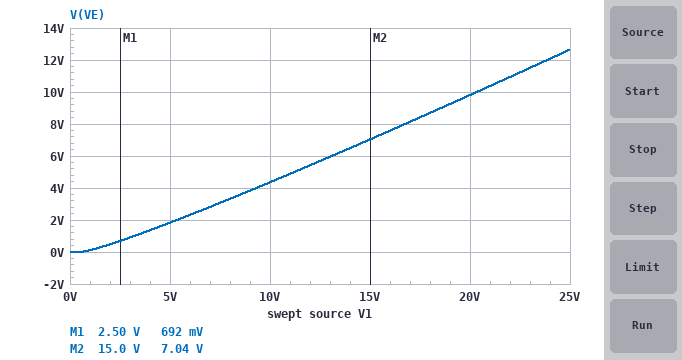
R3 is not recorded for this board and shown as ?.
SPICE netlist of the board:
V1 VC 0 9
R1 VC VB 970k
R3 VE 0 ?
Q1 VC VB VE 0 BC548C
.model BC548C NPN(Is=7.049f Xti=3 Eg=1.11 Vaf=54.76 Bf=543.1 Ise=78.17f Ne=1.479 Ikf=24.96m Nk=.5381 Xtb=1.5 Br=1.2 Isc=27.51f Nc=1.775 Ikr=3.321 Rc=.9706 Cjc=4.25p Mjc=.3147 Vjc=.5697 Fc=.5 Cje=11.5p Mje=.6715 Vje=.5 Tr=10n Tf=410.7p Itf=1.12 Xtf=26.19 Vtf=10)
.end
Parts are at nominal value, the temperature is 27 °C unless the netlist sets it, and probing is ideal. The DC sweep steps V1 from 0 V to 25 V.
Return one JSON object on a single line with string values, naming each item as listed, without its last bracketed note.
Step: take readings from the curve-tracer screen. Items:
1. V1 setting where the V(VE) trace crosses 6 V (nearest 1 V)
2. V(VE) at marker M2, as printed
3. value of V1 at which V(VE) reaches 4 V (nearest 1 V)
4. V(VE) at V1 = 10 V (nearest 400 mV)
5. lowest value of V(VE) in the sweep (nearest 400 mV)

{"V1 setting where the V(VE) trace crosses 6 V": "13 V", "V(VE) at marker M2, as printed": "7.04 V", "value of V1 at which V(VE) reaches 4 V": "9 V", "V(VE) at V1 = 10 V": "4.4 V", "lowest value of V(VE) in the sweep": "0 V"}
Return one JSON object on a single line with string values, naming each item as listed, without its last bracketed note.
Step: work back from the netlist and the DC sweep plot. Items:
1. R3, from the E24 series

{"R3, from the E24 series": "3.6 kΩ"}
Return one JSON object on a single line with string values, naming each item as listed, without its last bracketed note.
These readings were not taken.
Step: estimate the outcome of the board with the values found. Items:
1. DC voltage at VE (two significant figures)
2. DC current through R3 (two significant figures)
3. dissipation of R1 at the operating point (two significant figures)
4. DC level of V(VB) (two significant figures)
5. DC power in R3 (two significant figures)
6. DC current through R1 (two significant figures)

{"DC voltage at VE": "3.8 V", "DC current through R3": "1.1 mA", "dissipation of R1 at the operating point": "21 µW", "DC level of V(VB)": "4.5 V", "DC power in R3": "4.1 mW", "DC current through R1": "4.6 µA"}
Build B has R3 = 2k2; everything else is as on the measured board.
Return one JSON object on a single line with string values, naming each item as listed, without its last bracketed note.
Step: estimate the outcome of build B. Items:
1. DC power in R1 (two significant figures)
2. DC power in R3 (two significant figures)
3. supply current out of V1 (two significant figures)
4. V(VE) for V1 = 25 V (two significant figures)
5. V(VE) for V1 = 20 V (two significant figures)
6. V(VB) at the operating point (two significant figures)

{"DC power in R1": "30 µW", "DC power in R3": "3.9 mW", "supply current out of V1": "1.3 mA", "V(VE) for V1 = 25 V": "10 V", "V(VE) for V1 = 20 V": "7.7 V", "V(VB) at the operating point": "3.6 V"}
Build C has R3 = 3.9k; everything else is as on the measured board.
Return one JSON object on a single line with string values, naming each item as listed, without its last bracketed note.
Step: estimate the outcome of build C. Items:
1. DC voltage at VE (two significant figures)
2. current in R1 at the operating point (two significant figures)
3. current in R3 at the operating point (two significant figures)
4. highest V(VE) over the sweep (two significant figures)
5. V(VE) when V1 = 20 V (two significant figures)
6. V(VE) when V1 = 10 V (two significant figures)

{"DC voltage at VE": "4.0 V", "current in R1 at the operating point": "4.5 µA", "current in R3 at the operating point": "1.0 mA", "highest V(VE) over the sweep": "13 V", "V(VE) when V1 = 20 V": "10 V", "V(VE) when V1 = 10 V": "4.5 V"}
